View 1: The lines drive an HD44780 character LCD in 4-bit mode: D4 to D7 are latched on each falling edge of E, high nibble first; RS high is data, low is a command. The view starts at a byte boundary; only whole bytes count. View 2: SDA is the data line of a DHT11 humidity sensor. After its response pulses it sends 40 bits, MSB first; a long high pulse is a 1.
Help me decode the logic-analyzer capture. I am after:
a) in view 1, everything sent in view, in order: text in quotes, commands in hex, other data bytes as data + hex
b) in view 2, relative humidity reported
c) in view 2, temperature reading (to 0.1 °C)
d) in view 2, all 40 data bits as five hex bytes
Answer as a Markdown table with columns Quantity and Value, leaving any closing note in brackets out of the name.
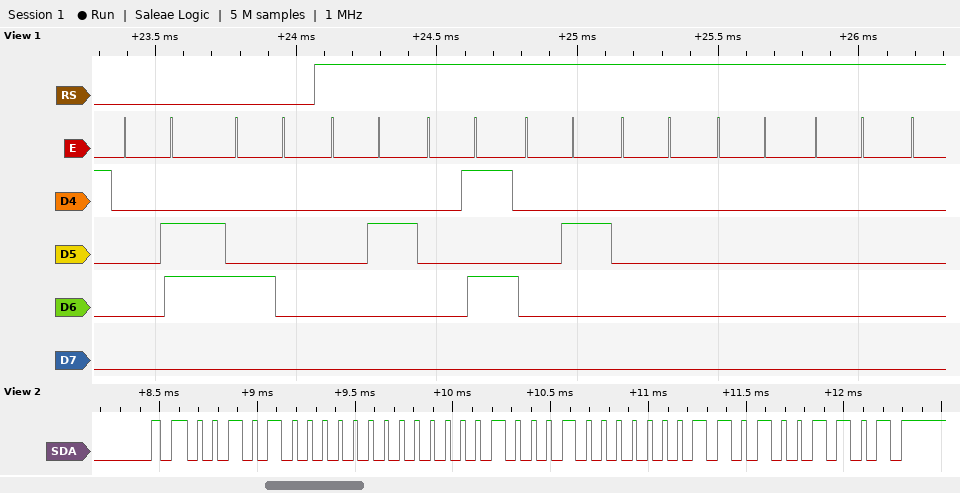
| Quantity | Value |
|---|---|
| in view 1, everything sent in view, in order: text in quotes, commands in hex, other data bytes as data + hex | 0x06 0x40 data 02 05 02 00 00 00 |
| in view 2, relative humidity reported | 40 % |
| in view 2, temperature reading | 34.3 °C |
| in view 2, all 40 data bits as five hex bytes | 28 00 22 03 4D |
